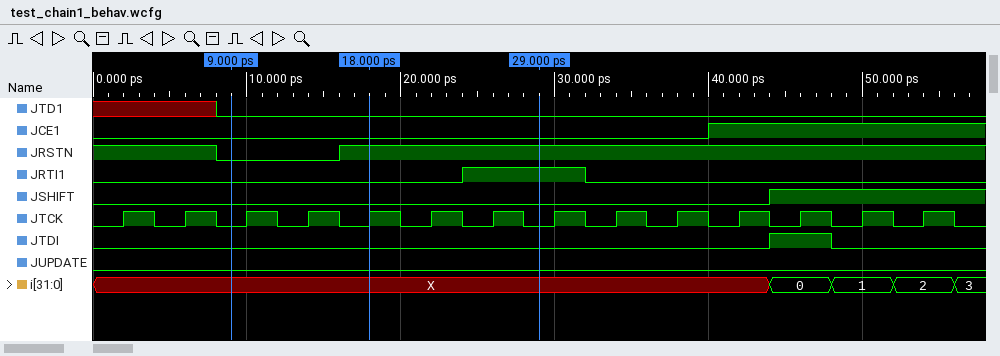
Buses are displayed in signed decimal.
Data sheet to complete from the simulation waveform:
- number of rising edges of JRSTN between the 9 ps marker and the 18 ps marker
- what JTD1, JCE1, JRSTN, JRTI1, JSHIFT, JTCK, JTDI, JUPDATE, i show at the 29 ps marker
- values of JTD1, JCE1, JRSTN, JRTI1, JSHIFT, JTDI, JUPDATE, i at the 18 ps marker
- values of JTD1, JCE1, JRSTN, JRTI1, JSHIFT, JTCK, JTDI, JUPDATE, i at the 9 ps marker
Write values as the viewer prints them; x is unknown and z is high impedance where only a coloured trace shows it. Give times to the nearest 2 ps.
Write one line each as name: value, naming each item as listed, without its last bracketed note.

number of rising edges of JRSTN between the 9 ps marker and the 18 ps marker: 1
what JTD1, JCE1, JRSTN, JRTI1, JSHIFT, JTCK, JTDI, JUPDATE, i show at the 29 ps marker: JTD1=0, JCE1=0, JRSTN=1, JRTI1=1, JSHIFT=0, JTCK=0, JTDI=0, JUPDATE=0, i=X
values of JTD1, JCE1, JRSTN, JRTI1, JSHIFT, JTDI, JUPDATE, i at the 18 ps marker: JTD1=0, JCE1=0, JRSTN=1, JRTI1=0, JSHIFT=0, JTDI=0, JUPDATE=0, i=X
values of JTD1, JCE1, JRSTN, JRTI1, JSHIFT, JTCK, JTDI, JUPDATE, i at the 9 ps marker: JTD1=0, JCE1=0, JRSTN=0, JRTI1=0, JSHIFT=0, JTCK=0, JTDI=0, JUPDATE=0, i=X
